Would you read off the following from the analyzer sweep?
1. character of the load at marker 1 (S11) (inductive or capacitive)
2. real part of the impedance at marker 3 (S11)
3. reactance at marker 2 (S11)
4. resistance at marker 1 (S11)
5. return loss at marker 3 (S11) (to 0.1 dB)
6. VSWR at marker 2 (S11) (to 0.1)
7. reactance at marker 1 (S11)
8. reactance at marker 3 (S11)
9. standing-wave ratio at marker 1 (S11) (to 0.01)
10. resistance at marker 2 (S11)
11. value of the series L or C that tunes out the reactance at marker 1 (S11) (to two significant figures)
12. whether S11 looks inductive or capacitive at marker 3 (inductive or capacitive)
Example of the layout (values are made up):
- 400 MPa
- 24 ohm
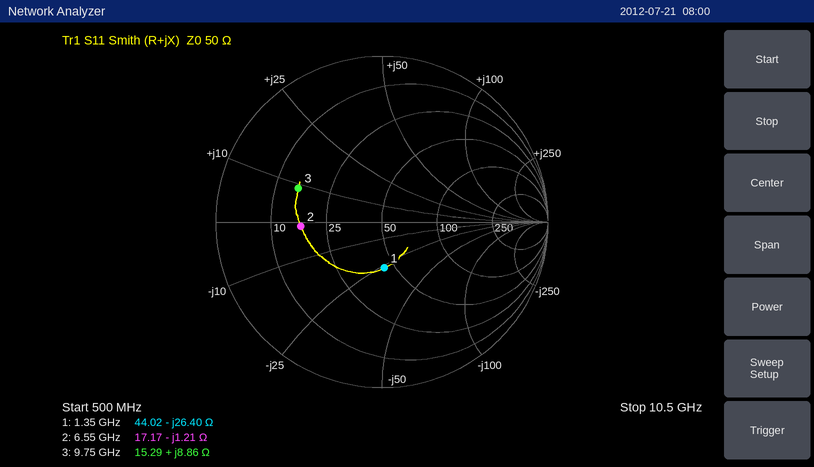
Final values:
- capacitive
- 15.29 Ω
- -1.21 Ω
- 44.02 Ω
- 5.3 dB
- 2.9
- -26.40 Ω
- +8.86 Ω
- 1.77
- 17.17 Ω
- 3.1 nH
- inductive
